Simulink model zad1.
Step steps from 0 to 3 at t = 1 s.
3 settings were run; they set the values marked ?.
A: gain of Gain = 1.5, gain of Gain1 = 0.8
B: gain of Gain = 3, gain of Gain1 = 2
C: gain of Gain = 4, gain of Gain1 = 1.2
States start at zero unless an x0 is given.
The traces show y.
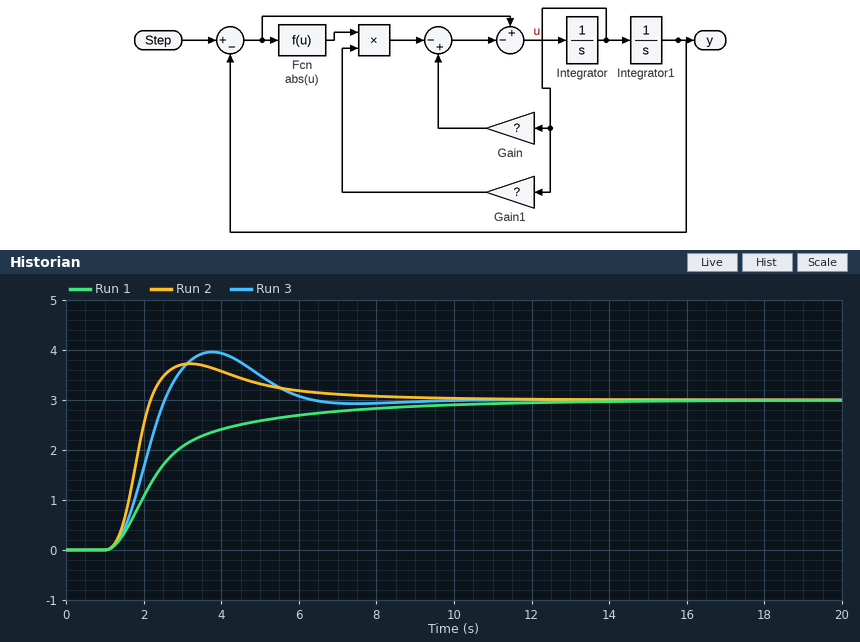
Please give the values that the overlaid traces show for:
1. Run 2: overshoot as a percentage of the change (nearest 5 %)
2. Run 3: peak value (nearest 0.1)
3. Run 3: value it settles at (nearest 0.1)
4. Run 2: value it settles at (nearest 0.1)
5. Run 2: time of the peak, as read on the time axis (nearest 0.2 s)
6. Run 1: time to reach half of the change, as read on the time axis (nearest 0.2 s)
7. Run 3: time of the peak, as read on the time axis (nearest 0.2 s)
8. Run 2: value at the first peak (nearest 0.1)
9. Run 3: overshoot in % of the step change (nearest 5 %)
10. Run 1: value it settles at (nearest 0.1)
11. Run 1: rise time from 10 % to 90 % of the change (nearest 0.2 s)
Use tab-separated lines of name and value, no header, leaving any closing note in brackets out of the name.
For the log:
Run 2: overshoot as a percentage of the change	25 %
Run 3: peak value	4.0
Run 3: value it settles at	3.0
Run 2: value it settles at	3.0
Run 2: time of the peak, as read on the time axis	3.2 s
Run 1: time to reach half of the change, as read on the time axis	2.4 s
Run 3: time of the peak, as read on the time axis	3.8 s
Run 2: value at the first peak	3.7
Run 3: overshoot in % of the step change	30 %
Run 1: value it settles at	3.0
Run 1: rise time from 10 % to 90 % of the change	4.6 s
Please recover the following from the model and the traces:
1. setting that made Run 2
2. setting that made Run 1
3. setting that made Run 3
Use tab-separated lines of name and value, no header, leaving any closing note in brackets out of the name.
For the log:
setting that made Run 2	B
setting that made Run 1	C
setting that made Run 3	A
